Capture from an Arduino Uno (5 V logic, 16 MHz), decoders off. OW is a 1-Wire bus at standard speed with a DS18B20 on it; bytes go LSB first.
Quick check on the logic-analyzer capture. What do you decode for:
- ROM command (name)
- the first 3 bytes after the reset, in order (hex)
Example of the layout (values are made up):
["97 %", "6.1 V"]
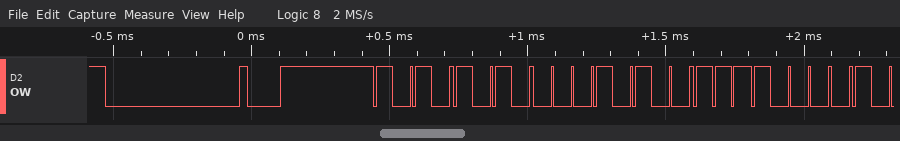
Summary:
["Match ROM", "55 28 0F"]
